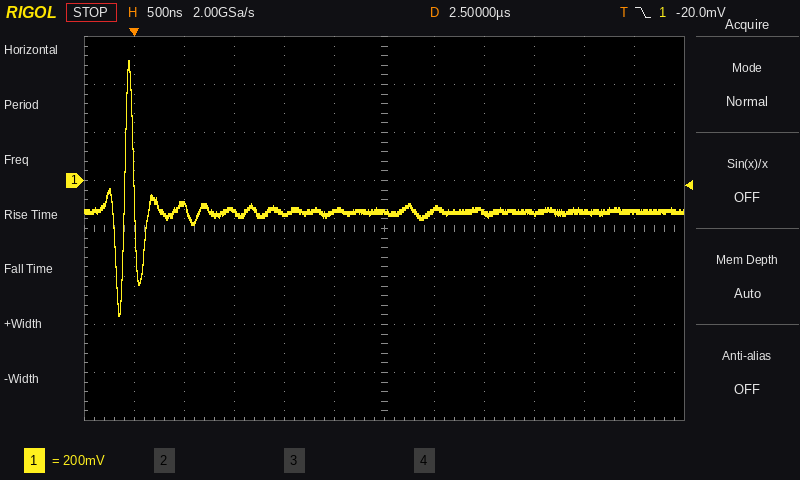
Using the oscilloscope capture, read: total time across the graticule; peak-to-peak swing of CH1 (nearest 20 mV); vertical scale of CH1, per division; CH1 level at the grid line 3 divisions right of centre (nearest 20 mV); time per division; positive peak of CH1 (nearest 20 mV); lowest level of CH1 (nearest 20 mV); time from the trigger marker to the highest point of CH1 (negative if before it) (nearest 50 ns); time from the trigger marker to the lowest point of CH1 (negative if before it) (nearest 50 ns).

6 µs
1.06 V
200 mV
-140 mV
500 ns
500 mV
-560 mV
-50 ns
-150 ns
